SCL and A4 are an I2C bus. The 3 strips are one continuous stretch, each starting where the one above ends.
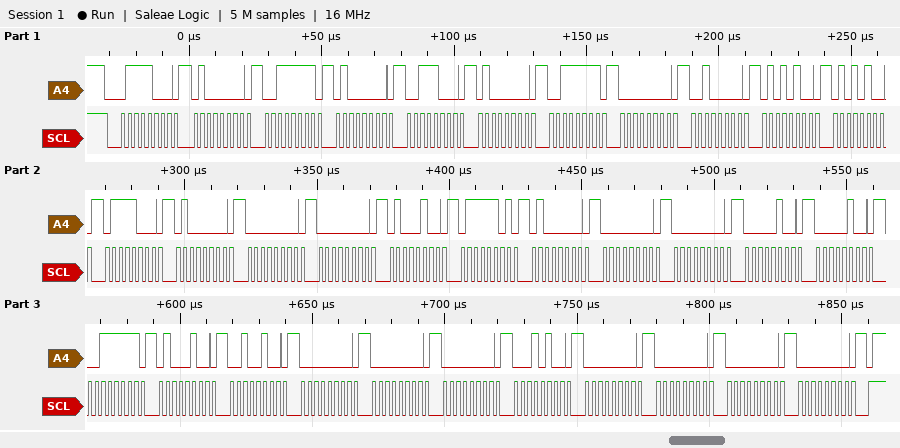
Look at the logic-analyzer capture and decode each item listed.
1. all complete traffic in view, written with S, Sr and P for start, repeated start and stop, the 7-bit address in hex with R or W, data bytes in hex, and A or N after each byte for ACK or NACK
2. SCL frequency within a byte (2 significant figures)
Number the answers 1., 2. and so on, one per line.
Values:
1. S 3CW A 40 A 3F A 40 A 38 A 40 A 3F A 00 A 20 A 54 A 54 A 78 A 40 A 00 A 00 A 44 A 7D A 40 A 00 A 00 A 04 A 04 A 3F A 44 A 24 A 00 A 00 A 00 A 14 A 00 A 00 A 00 A 00 A P
2. 400 kHz
